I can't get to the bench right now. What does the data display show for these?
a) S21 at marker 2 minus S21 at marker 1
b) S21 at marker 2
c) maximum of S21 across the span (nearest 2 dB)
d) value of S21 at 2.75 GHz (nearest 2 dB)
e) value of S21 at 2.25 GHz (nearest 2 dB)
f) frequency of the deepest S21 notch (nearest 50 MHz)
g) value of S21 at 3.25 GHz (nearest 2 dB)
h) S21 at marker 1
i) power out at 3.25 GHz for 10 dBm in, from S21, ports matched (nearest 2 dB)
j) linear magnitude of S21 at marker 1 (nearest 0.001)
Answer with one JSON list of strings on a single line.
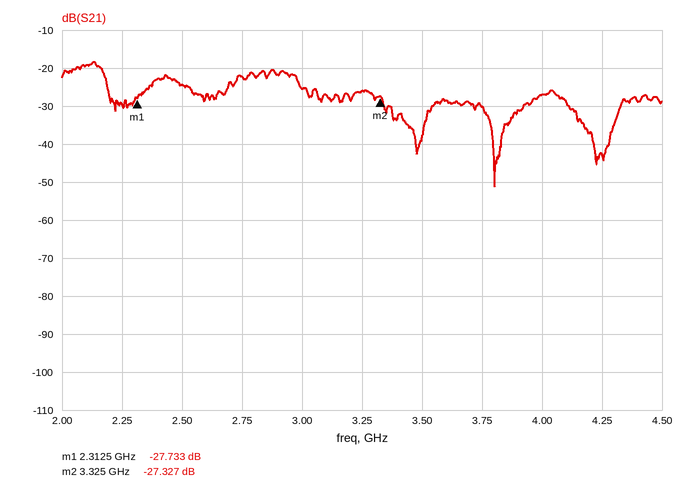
["0.406 dB", "-27.327 dB", "-18 dB", "-22 dB", "-30 dB", "3.80 GHz", "-26 dB", "-27.733 dB", "-16 dBm", "0.041"]
